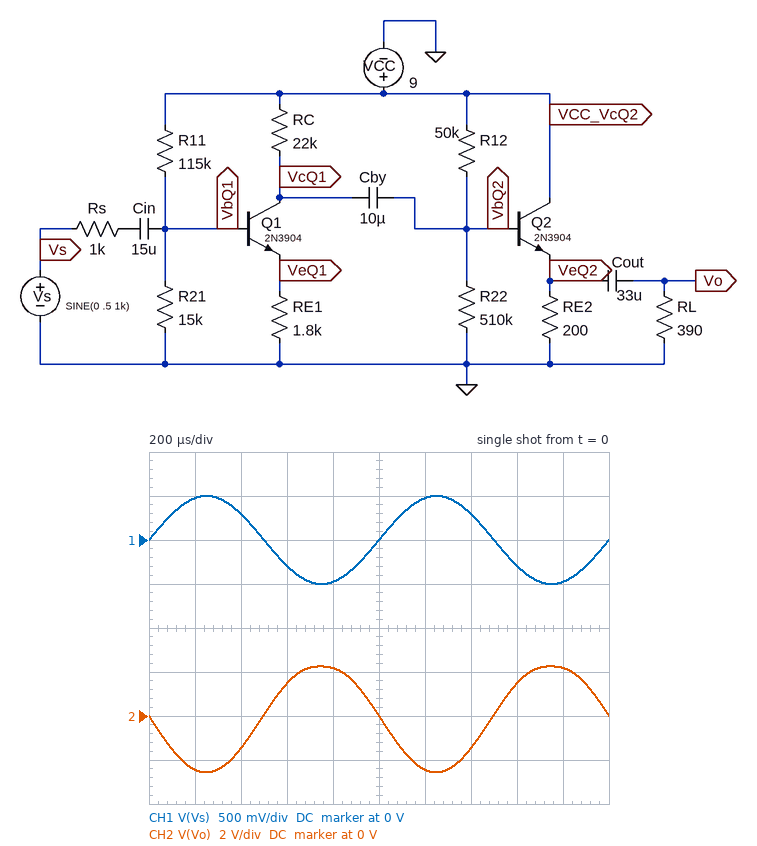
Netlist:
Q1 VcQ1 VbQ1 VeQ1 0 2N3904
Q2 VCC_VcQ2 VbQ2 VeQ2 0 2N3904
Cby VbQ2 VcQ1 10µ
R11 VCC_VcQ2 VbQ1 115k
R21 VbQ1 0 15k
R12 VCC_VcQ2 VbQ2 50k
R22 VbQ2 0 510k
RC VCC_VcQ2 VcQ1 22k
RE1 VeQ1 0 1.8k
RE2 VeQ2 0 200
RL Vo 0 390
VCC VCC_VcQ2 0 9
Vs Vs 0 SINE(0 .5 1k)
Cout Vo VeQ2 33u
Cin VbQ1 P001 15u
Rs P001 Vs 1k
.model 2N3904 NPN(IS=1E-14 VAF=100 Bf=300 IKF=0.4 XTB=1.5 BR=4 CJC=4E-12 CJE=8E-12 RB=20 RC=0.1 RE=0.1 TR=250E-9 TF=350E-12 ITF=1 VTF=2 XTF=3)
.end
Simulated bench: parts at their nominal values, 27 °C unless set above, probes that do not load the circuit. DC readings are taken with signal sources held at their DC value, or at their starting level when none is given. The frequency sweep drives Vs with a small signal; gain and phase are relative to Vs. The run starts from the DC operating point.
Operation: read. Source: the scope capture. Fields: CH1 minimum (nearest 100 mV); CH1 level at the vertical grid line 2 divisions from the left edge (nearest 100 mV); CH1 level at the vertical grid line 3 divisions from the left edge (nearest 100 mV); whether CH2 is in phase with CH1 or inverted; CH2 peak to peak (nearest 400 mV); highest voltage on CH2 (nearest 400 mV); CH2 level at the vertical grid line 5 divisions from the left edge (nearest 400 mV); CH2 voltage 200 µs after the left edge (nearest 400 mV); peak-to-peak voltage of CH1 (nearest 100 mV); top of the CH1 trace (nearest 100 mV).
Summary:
-500 mV
300 mV
-300 mV
inverted
4.8 V
2.4 V
0 V
-2.4 V
1.0 V
500 mV
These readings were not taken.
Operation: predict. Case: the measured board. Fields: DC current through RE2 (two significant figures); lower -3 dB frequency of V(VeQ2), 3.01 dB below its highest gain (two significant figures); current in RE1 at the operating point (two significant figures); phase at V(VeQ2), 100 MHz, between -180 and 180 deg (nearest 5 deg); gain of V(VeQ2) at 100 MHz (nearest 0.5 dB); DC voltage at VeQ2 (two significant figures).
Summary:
21 mA
840 mHz
230 µA
-25 deg
-14.0 dB
4.2 V
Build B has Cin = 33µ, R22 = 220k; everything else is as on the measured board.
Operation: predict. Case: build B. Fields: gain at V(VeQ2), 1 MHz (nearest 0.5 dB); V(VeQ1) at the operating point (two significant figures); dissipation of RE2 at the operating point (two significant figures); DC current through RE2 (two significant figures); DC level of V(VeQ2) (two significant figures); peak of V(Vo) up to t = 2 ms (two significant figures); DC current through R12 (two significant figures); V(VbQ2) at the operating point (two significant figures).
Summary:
12.5 dB
410 mV
77 mW
20 mA
3.9 V
2.2 V
87 µA
4.7 V
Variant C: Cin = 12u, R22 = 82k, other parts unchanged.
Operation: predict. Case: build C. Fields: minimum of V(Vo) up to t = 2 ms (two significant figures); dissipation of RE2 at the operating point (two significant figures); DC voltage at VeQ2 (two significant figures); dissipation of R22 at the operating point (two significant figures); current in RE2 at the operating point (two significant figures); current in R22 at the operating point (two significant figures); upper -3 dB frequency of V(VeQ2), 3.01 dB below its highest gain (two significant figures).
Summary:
-2.1 V
52 mW
3.2 V
190 µW
16 mA
48 µA
1.7 MHz
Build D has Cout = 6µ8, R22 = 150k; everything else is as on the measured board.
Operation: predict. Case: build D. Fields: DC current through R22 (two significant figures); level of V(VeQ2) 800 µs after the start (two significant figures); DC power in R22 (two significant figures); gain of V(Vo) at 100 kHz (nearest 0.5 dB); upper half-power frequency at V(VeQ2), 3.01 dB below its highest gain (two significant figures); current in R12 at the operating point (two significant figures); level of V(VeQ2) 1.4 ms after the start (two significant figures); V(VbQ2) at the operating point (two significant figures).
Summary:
30 µA
5.8 V
130 µW
13.5 dB
1.5 MHz
91 µA
2.2 V
4.4 V
